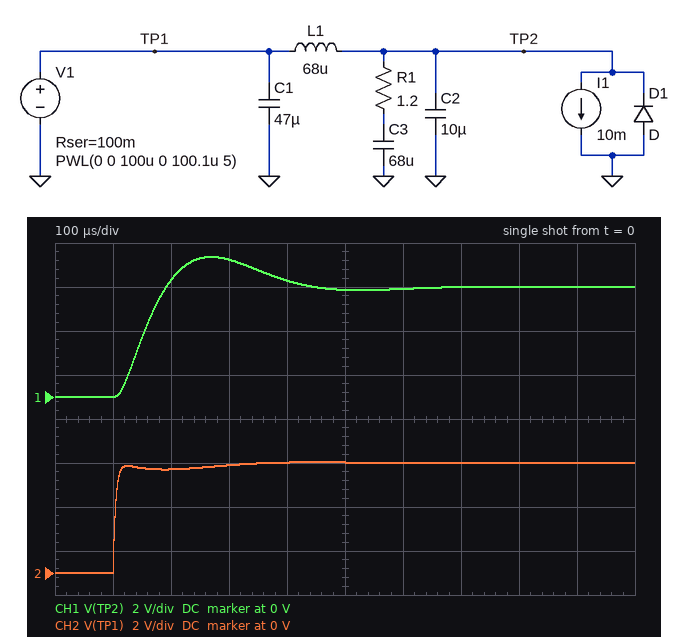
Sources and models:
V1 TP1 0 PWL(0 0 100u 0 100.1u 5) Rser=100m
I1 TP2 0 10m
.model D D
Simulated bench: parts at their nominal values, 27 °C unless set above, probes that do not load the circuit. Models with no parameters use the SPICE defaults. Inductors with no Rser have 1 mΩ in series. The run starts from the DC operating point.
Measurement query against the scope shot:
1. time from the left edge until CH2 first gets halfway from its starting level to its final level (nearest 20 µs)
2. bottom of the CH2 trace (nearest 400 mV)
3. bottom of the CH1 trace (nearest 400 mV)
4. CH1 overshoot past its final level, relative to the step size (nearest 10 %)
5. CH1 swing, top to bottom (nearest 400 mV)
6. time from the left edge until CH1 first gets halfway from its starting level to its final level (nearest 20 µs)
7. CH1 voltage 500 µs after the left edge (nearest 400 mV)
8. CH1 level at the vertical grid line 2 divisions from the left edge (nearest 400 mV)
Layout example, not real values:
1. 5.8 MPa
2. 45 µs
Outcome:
1. 100 µs
2. 0 V
3. 0 V
4. 30 %
5. 6.4 V
6. 140 µs
7. 4.8 V
8. 5.2 V
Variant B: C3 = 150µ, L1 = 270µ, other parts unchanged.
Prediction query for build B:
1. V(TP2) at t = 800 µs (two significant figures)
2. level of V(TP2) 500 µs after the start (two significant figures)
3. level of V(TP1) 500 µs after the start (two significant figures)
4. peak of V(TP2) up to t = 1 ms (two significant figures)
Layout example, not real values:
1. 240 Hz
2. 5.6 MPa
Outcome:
1. 6.1 V
2. 6.3 V
3. 4.8 V
4. 6.6 V
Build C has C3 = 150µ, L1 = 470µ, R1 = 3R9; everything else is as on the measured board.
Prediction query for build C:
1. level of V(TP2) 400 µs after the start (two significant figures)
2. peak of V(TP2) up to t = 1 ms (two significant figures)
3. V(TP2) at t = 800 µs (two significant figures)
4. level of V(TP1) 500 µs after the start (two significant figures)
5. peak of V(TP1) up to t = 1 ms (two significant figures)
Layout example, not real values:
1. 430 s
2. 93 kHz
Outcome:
1. 5.4 V
2. 5.7 V
3. 5.5 V
4. 4.9 V
5. 5.0 V
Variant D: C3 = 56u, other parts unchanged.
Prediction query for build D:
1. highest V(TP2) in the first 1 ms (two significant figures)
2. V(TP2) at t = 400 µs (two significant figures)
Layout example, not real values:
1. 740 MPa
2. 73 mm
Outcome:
1. 6.6 V
2. 5.1 V
